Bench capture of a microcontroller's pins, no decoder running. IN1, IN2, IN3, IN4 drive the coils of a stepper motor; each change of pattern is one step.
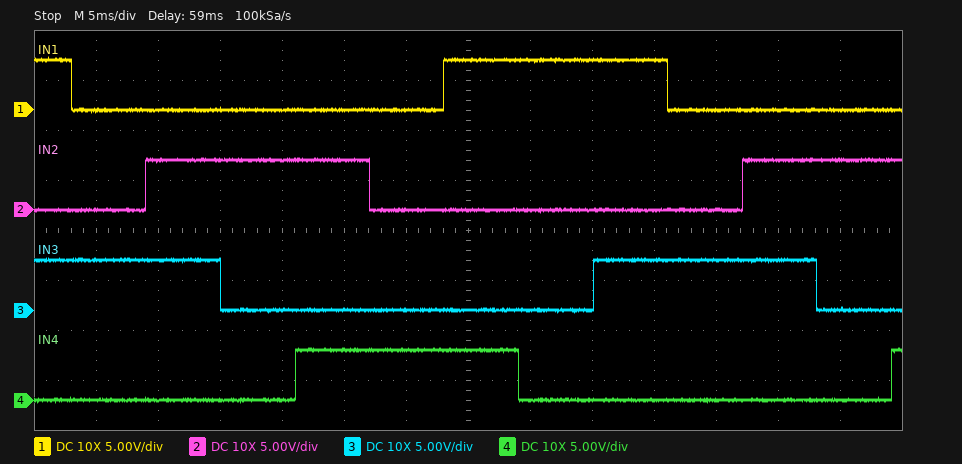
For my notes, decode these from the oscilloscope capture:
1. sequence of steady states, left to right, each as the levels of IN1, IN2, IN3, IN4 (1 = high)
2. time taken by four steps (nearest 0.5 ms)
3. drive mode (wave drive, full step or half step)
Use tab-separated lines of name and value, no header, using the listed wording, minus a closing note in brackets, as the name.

sequence of steady states, left to right, each as the levels of IN1, IN2, IN3, IN4	1010 0010 0110 0100 0101 0001 1001 1000 1010 0010 0110 0100 0101
time taken by four steps	24.0 ms
drive mode	half step
